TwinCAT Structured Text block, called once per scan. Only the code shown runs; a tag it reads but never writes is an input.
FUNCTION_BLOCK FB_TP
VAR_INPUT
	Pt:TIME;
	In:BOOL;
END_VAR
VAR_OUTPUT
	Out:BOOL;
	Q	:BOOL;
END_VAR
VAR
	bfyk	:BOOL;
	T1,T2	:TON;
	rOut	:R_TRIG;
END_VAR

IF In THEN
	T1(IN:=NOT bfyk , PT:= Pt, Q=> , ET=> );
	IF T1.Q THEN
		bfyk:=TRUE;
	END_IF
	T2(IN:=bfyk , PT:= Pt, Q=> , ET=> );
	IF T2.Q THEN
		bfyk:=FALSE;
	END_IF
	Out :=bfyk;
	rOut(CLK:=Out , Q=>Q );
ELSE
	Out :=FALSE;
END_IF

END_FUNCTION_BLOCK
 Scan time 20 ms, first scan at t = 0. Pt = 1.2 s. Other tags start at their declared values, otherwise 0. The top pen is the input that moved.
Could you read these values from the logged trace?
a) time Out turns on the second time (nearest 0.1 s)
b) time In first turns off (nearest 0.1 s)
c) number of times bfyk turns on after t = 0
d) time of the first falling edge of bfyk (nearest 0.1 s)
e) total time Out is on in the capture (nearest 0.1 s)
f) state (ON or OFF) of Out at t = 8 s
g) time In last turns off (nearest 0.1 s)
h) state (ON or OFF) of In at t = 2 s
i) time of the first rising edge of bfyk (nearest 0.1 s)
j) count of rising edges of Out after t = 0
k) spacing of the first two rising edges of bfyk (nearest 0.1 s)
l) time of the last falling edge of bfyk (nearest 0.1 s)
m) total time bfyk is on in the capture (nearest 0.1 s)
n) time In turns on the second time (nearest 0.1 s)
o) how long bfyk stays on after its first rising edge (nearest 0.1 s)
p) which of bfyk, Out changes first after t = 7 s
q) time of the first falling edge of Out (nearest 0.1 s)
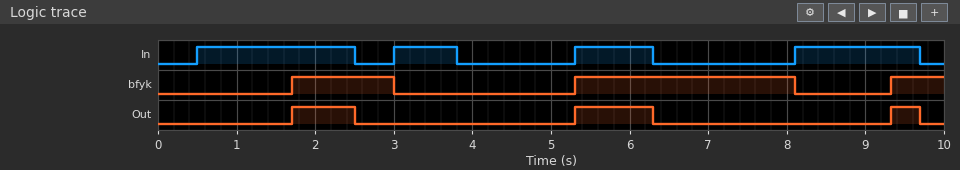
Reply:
5.3 s
2.5 s
3
3.0 s
2.2 s
OFF
9.7 s
ON
1.7 s
3
3.6 s
8.1 s
4.8 s
3.0 s
1.3 s
bfyk
2.5 s
